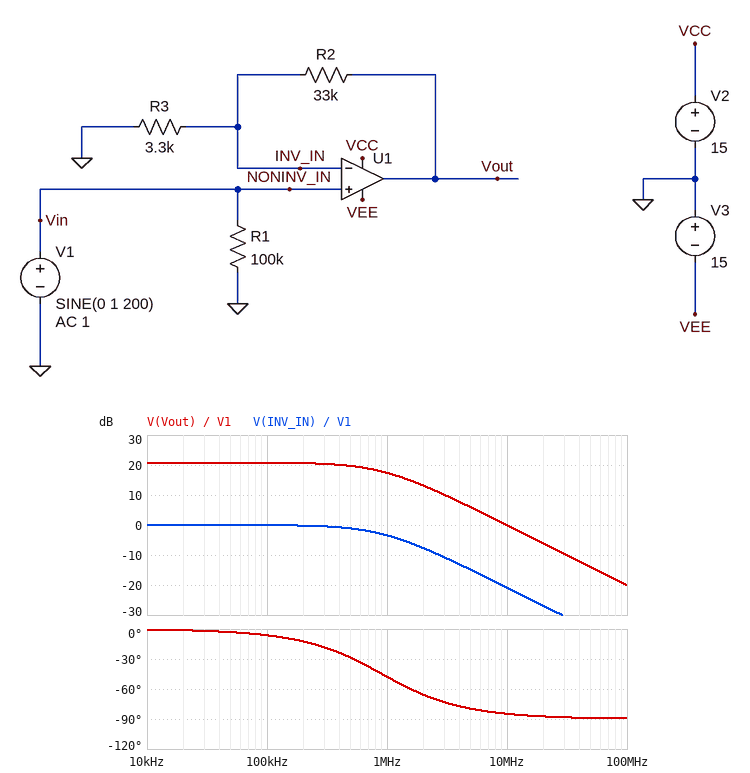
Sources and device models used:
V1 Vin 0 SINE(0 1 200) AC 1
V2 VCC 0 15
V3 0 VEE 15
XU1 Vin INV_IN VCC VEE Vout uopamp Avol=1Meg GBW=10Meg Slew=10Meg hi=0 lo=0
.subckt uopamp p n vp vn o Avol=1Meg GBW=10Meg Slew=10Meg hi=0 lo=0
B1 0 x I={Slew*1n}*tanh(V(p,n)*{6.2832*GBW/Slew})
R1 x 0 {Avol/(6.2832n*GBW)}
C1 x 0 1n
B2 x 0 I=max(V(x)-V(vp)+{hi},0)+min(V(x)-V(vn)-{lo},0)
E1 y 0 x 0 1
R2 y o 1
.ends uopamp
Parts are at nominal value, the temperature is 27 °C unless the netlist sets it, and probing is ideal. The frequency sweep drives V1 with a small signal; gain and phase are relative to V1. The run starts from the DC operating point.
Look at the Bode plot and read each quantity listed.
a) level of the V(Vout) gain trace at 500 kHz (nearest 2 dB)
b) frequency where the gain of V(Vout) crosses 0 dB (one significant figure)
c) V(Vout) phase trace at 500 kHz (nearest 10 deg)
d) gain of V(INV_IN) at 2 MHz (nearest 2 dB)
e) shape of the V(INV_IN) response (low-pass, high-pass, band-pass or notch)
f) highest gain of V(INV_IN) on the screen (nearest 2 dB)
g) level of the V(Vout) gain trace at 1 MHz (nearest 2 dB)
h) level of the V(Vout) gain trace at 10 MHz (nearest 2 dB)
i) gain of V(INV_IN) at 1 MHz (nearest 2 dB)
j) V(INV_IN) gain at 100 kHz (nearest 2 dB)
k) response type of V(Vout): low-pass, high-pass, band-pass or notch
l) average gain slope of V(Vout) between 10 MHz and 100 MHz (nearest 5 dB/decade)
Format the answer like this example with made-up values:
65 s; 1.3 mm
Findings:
20 dB; 10 MHz; -30 deg; -8 dB; low-pass; 0 dB; 18 dB; 0 dB; -4 dB; 0 dB; low-pass; -20 dB/decade
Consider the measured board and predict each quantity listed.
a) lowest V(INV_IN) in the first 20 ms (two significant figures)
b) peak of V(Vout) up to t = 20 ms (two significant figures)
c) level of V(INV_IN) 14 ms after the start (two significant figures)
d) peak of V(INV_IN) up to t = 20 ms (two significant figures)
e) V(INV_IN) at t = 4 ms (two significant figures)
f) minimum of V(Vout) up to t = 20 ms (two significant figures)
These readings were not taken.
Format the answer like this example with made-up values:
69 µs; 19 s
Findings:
-1.0 V; 11 V; -950 mV; 1.0 V; -950 mV; -11 V
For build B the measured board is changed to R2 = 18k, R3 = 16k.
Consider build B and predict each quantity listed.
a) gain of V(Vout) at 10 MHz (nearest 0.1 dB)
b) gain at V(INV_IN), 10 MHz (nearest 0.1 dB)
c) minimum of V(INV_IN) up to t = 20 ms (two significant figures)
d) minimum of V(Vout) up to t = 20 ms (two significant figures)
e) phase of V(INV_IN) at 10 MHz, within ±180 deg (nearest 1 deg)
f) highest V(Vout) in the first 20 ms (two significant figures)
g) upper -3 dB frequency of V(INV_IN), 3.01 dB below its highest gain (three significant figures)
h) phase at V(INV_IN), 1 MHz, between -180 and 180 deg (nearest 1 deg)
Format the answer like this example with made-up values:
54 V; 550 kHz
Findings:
-0.9 dB; -7.4 dB; -1.0 V; -2.1 V; -65 deg; 2.1 V; 4.71 MHz; -12 deg
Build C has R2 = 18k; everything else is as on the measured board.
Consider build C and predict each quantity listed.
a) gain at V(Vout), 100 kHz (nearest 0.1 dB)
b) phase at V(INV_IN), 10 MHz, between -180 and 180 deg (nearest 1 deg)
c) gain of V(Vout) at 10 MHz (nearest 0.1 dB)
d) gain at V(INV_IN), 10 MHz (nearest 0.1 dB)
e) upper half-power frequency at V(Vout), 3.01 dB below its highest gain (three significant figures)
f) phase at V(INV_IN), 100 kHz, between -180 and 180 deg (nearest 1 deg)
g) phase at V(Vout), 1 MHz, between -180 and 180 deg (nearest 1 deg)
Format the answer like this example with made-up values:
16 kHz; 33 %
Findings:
16.2 dB; -81 deg; -0.1 dB; -16.3 dB; 1.55 MHz; -4 deg; -33 deg
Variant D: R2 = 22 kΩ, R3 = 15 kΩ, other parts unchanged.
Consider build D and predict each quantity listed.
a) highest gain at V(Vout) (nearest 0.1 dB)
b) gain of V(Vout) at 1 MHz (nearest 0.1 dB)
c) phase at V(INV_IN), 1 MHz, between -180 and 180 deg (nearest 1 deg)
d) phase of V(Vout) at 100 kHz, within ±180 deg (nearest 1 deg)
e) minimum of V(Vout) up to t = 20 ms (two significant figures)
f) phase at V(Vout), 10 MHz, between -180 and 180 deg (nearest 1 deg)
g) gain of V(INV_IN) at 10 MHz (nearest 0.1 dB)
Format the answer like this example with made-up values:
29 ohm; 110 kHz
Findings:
7.8 dB; 7.6 dB; -14 deg; -1 deg; -2.5 V; -68 deg; -8.5 dB
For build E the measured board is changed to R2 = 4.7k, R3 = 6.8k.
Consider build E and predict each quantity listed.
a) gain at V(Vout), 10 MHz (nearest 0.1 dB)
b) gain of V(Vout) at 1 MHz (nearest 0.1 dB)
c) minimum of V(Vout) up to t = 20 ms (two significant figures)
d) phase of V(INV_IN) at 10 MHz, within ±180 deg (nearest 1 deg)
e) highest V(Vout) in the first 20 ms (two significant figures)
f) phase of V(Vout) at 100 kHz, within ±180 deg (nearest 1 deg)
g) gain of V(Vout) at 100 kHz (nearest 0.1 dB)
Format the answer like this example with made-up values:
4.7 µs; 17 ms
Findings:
-1.3 dB; 4.4 dB; -1.7 V; -59 deg; 1.7 V; -1 deg; 4.6 dB
